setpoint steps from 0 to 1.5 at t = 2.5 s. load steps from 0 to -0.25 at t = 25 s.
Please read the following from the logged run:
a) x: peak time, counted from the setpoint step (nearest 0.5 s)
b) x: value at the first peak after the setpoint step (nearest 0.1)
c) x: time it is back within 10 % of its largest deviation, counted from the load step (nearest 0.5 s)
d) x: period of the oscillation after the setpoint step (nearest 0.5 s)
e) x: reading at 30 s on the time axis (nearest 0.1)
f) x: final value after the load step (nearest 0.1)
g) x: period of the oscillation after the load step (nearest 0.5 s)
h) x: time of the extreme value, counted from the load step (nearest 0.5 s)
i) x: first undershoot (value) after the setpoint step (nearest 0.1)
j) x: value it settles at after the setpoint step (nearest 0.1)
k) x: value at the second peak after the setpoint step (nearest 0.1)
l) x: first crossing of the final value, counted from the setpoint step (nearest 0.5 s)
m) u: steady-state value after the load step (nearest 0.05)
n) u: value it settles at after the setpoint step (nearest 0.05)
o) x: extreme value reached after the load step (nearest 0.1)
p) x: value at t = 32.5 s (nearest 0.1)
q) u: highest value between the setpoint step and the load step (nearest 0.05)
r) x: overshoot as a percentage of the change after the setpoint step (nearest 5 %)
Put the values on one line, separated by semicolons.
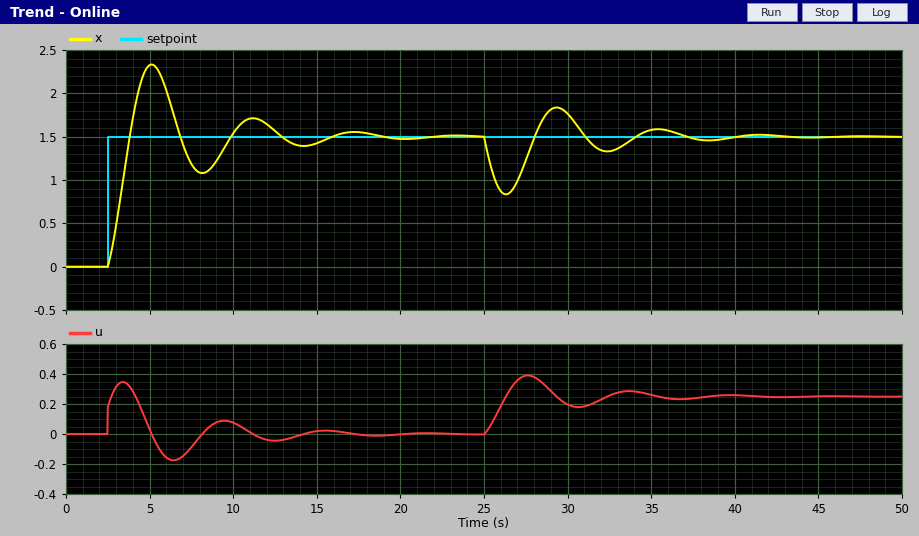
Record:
2.5 s; 2.3; 11.0 s; 6.0 s; 1.8; 1.5; 6.0 s; 1.5 s; 1.1; 1.5; 1.7; 1.5 s; 0.25; 0.00; 0.8; 1.3; 0.35; 55 %
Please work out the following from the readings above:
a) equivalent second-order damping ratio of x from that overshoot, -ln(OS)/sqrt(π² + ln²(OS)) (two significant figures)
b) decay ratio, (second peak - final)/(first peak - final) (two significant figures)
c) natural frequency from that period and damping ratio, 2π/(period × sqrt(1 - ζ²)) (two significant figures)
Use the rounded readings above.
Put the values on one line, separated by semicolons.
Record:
0.19; 0.25; 1.1 rad/s
